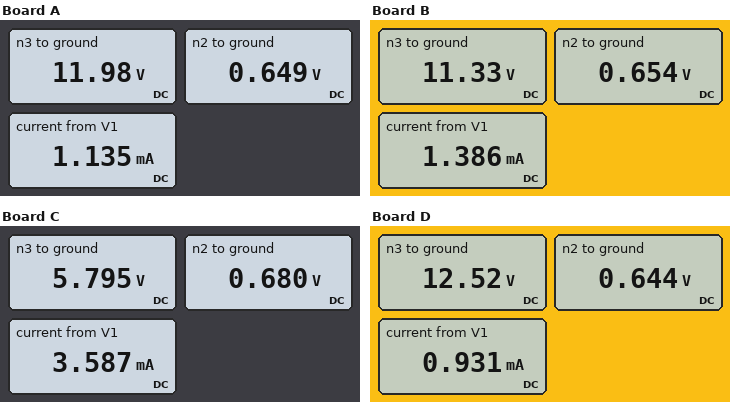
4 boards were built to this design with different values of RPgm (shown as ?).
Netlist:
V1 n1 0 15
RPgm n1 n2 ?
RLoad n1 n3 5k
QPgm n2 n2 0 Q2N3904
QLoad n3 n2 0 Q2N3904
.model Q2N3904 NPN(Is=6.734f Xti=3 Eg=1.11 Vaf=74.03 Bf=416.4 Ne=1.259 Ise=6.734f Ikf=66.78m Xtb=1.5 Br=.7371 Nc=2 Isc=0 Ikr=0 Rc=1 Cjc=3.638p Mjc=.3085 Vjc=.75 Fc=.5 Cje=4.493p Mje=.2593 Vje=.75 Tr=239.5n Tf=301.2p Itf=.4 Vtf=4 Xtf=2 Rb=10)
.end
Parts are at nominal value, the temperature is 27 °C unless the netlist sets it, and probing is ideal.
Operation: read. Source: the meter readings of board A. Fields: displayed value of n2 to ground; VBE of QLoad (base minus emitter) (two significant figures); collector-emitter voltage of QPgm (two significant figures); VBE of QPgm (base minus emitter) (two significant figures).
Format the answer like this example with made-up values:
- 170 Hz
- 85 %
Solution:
- 0.649 V
- 650 mV
- 650 mV
- 650 mV
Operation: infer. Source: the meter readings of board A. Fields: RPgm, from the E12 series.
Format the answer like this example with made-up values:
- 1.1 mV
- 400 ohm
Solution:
- 27 kΩ
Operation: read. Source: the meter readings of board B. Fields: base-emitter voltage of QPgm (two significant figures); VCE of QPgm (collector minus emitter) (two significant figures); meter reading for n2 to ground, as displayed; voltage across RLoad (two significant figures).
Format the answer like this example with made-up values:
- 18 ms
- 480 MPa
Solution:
- 650 mV
- 650 mV
- 0.654 V
- 3.7 V
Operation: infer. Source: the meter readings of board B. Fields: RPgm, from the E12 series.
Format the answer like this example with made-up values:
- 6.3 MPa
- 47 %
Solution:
- 22 kΩ
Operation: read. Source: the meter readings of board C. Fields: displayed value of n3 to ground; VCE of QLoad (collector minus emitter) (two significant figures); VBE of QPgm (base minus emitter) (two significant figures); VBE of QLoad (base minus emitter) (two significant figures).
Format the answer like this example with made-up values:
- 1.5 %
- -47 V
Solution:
- 5.795 V
- 5.8 V
- 680 mV
- 680 mV
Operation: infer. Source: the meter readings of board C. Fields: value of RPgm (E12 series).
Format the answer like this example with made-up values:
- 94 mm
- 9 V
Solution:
- 8.2 kΩ
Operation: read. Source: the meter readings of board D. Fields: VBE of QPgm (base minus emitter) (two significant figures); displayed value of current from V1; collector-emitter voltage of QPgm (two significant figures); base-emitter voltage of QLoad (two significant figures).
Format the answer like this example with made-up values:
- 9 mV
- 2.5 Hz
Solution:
- 640 mV
- 0.931 mA
- 640 mV
- 640 mV
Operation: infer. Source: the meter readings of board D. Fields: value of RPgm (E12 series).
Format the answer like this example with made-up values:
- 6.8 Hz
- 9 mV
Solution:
- 33 kΩ
